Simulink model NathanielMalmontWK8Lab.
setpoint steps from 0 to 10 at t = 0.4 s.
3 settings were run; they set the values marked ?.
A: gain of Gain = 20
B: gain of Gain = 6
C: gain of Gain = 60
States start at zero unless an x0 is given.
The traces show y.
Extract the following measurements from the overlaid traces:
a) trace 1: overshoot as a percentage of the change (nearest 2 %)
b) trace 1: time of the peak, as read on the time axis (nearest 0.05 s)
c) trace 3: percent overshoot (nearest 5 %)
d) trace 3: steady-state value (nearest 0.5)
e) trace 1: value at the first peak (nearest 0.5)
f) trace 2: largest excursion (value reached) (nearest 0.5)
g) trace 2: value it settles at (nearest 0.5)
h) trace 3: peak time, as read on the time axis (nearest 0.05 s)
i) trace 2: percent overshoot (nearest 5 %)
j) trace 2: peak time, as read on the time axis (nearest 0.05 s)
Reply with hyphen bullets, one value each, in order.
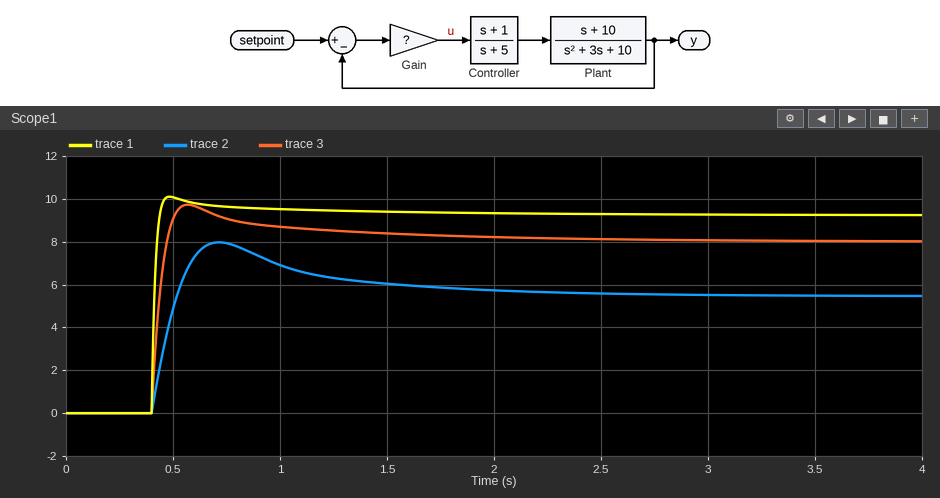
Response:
- 10 %
- 0.50 s
- 20 %
- 8.0
- 10.0
- 8.0
- 5.5
- 0.55 s
- 45 %
- 0.70 s
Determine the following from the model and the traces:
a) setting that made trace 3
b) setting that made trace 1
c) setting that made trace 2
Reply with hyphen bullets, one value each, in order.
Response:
- A
- C
- B
